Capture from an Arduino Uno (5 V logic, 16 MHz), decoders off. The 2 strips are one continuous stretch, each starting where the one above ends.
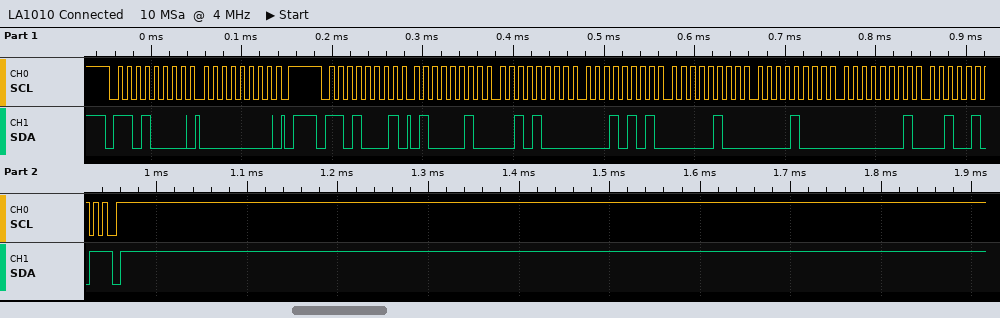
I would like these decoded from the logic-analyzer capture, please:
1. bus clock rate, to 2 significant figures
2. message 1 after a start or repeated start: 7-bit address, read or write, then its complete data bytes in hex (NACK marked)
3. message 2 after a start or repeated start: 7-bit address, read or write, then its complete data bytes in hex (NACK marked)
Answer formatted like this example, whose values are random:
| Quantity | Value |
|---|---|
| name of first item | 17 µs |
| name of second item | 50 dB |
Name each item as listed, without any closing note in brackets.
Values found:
| Quantity | Value |
|---|---|
| bus clock rate, to 2 significant figures | 100 kHz |
| message 1 after a start or repeated start: 7-bit address, read or write, then its complete data bytes in hex | 0x68 write: 00 |
| message 2 after a start or repeated start: 7-bit address, read or write, then its complete data bytes in hex | 0x68 read: 42 28 15 04 08 01 25 NACK |
